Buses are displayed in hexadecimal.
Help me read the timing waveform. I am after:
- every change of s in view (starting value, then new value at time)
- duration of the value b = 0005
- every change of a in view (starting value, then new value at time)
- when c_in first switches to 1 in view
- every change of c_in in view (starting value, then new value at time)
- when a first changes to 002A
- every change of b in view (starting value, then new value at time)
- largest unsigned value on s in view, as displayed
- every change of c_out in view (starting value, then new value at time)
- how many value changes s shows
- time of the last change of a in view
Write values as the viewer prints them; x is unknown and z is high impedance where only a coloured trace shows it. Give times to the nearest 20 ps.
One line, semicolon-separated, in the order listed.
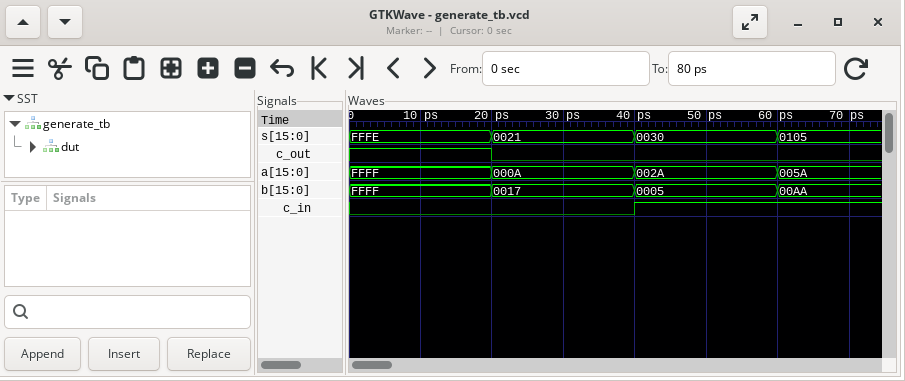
FFFE, 0021 at 20 ps, 0030 at 40 ps, 0105 at 60 ps; 20 ps; FFFF, 000A at 20 ps, 002A at 40 ps, 005A at 60 ps; 40 ps; 0, 1 at 40 ps; 40 ps; FFFF, 0017 at 20 ps, 0005 at 40 ps, 00AA at 60 ps; FFFE; 1, 0 at 20 ps; 3; 60 ps
